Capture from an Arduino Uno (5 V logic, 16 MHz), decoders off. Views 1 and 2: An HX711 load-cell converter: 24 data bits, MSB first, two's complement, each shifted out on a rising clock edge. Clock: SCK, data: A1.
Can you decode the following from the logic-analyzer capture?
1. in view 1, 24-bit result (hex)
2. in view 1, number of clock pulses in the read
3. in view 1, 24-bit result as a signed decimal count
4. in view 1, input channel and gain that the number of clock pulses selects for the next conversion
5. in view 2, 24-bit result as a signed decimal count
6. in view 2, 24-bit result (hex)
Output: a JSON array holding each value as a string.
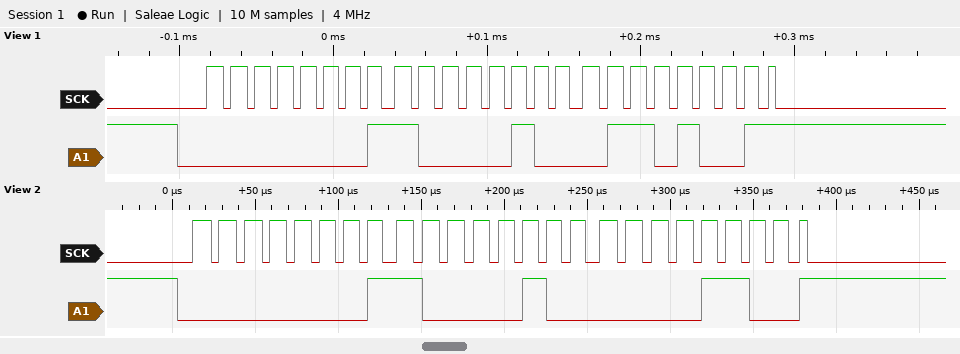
["0x018469", "25", "99433", "channel A, gain 128", "99340", "0x01840C"]
